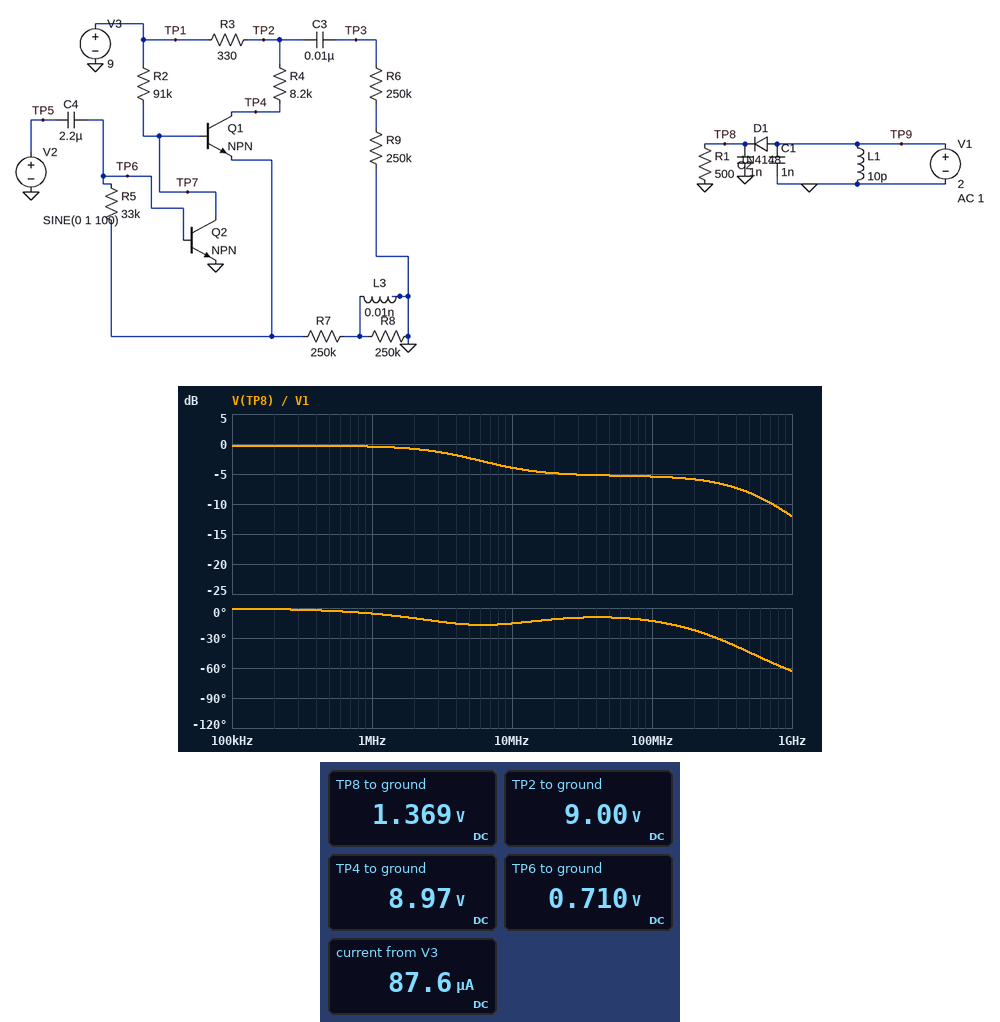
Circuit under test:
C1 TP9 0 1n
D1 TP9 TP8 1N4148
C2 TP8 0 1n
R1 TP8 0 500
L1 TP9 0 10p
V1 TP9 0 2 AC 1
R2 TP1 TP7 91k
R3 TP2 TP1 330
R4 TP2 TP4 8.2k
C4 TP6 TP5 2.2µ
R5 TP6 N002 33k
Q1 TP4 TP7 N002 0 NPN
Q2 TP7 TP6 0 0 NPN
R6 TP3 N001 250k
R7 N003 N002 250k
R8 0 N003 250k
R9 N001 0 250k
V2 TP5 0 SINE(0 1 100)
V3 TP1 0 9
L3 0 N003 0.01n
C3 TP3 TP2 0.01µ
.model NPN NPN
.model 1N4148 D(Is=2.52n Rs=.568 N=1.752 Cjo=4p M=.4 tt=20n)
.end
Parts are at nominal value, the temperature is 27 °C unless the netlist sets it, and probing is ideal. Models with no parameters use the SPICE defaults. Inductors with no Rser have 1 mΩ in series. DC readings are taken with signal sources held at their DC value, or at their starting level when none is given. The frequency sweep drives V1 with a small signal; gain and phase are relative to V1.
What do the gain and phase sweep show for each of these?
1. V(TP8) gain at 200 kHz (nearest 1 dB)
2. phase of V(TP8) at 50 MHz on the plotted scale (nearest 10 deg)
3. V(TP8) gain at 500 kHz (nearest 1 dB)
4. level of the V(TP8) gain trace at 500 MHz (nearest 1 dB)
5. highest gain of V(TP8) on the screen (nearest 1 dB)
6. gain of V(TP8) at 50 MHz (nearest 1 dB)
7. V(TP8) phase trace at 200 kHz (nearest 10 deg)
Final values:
0 dB
-10 deg
0 dB
-8 dB
0 dB
-5 dB
0 deg
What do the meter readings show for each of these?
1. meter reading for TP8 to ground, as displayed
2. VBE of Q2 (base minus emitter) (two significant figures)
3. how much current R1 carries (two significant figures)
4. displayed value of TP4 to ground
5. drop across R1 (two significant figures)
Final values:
1.369 V
710 mV
2.7 mA
8.97 V
1.4 V
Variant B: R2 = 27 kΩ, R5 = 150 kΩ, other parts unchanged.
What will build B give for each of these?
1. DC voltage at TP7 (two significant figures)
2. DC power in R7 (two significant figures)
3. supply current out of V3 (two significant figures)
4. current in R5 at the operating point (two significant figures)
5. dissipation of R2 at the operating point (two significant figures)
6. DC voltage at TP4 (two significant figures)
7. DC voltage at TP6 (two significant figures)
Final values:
1.8 V
5.2 µW
270 µA
2.7 µA
1.9 mW
8.9 V
740 mV
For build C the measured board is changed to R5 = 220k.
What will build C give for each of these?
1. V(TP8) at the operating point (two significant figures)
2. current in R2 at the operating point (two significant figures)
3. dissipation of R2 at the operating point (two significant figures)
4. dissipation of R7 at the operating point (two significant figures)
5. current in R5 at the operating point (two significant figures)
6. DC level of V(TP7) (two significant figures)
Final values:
1.4 V
82 µA
610 µW
3.2 µW
820 nA
1.5 V
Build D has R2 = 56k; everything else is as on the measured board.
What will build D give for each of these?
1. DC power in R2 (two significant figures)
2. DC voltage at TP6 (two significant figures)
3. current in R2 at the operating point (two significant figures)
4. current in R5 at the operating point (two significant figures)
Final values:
1.0 mW
720 mV
140 µA
1.4 µA
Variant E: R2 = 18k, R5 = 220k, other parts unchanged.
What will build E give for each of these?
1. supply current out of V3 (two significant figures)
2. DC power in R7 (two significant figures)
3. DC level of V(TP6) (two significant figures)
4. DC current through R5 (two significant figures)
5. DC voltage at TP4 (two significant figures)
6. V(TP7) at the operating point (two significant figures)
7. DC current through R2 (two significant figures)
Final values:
390 µA
9.9 µW
750 mV
3.8 µA
8.9 V
2.2 V
380 µA
